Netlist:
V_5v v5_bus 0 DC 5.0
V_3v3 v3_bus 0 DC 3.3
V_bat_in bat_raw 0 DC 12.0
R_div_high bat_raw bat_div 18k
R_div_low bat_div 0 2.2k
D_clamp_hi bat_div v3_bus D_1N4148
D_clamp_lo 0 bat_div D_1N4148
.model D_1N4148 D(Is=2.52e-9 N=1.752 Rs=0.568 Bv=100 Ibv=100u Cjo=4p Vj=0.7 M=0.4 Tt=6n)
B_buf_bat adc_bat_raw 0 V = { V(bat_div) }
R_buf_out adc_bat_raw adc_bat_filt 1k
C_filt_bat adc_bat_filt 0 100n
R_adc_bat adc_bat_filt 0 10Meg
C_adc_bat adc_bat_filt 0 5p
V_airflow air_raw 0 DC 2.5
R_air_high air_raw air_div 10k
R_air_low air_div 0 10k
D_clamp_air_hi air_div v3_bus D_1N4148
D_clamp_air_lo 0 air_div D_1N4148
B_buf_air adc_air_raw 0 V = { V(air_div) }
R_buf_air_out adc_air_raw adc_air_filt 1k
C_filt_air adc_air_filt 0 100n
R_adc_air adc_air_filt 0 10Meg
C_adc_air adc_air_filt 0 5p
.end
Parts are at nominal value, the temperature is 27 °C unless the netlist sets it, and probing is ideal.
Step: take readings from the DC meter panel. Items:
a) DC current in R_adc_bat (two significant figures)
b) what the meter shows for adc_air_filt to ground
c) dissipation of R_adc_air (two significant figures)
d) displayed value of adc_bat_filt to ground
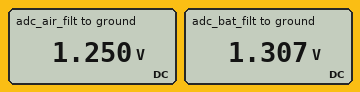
130 nA
1.250 V
160 nW
1.307 V
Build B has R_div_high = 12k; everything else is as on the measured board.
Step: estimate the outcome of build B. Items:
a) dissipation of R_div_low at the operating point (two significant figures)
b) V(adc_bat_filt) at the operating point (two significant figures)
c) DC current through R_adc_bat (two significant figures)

1.6 mW
1.9 V
190 nA
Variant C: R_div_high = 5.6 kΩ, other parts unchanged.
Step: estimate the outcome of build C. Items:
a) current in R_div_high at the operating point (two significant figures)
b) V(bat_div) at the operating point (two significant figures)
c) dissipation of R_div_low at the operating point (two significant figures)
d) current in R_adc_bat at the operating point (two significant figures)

1.5 mA
3.4 V
5.2 mW
340 nA
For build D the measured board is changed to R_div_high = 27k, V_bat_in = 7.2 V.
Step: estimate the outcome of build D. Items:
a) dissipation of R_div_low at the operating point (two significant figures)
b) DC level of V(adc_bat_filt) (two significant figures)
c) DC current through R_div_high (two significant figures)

130 µW
540 mV
250 µA
